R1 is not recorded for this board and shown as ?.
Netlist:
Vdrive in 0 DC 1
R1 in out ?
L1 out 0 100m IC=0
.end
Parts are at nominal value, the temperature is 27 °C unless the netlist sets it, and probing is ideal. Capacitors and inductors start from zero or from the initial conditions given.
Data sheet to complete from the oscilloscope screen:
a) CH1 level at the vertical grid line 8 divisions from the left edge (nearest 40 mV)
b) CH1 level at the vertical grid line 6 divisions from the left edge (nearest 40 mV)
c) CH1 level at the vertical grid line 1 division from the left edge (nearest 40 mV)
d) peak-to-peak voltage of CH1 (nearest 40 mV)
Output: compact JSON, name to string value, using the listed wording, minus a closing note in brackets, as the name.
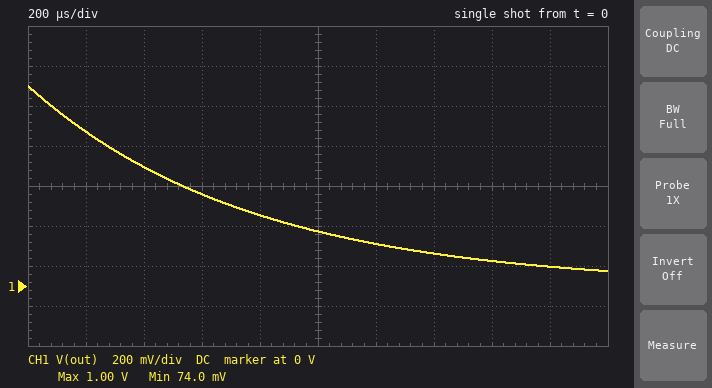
{"CH1 level at the vertical grid line 8 divisions from the left edge": "120 mV", "CH1 level at the vertical grid line 6 divisions from the left edge": "200 mV", "CH1 level at the vertical grid line 1 division from the left edge": "760 mV", "peak-to-peak voltage of CH1": "920 mV"}
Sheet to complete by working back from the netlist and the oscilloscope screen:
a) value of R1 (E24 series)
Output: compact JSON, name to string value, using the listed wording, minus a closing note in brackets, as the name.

{"value of R1": "130 Ω"}
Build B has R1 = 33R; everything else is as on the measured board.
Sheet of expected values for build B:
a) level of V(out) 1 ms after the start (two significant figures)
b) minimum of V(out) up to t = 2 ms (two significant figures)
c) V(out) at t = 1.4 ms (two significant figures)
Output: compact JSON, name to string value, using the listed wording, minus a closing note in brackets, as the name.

{"level of V(out) 1 ms after the start": "720 mV", "minimum of V(out) up to t = 2 ms": "520 mV", "V(out) at t = 1.4 ms": "630 mV"}
